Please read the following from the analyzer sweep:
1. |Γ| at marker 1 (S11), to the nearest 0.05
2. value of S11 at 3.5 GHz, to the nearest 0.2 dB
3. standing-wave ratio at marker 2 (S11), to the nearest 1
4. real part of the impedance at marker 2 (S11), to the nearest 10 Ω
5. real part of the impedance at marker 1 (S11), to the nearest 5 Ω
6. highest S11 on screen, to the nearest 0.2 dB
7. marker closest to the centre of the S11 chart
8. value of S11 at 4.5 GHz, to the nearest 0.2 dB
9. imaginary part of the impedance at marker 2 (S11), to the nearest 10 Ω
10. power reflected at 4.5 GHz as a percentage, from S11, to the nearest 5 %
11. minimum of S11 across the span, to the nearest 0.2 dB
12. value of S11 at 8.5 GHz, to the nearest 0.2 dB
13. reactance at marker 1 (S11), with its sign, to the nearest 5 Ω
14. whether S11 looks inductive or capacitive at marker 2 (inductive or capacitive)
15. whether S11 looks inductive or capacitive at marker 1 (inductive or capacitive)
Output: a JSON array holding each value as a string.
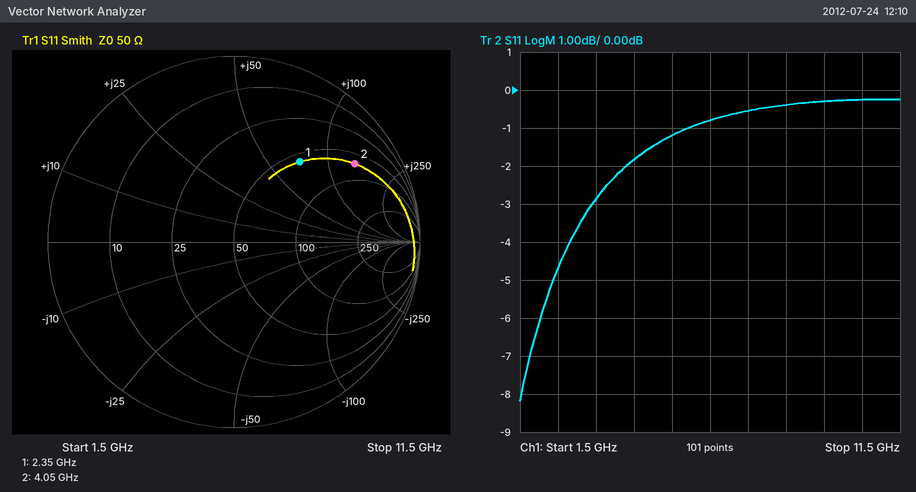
["0.55", "-2.8 dB", "8", "70 Ω", "55 Ω", "-0.2 dB", "marker 1", "-1.8 dB", "+140 Ω", "65 %", "-8.2 dB", "-0.4 dB", "+70 Ω", "inductive", "inductive"]
